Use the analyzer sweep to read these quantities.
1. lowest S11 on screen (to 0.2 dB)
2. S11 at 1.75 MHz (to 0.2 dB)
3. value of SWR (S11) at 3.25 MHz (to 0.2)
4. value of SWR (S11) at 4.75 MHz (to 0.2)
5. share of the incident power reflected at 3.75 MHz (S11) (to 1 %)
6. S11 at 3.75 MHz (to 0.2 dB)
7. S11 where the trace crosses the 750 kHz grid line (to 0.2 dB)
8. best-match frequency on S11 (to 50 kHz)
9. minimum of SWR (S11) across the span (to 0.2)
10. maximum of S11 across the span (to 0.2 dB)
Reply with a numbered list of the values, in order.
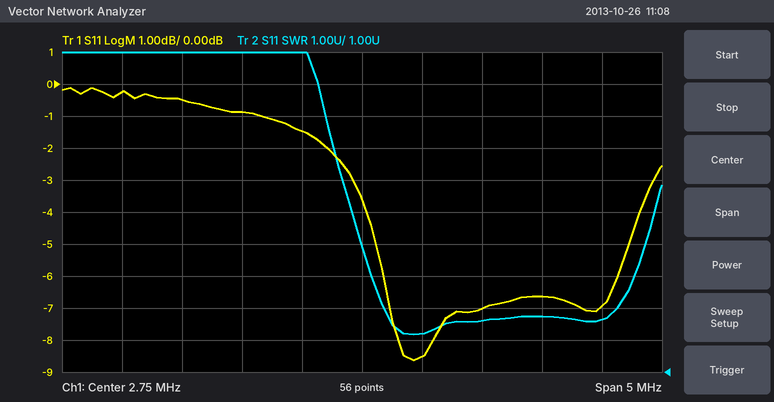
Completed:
1. -8.6 dB
2. -0.8 dB
3. 2.2
4. 2.6
5. 20 %
6. -7.0 dB
7. -0.2 dB
8. 3.20 MHz
9. 2.2
10. -0.2 dB
